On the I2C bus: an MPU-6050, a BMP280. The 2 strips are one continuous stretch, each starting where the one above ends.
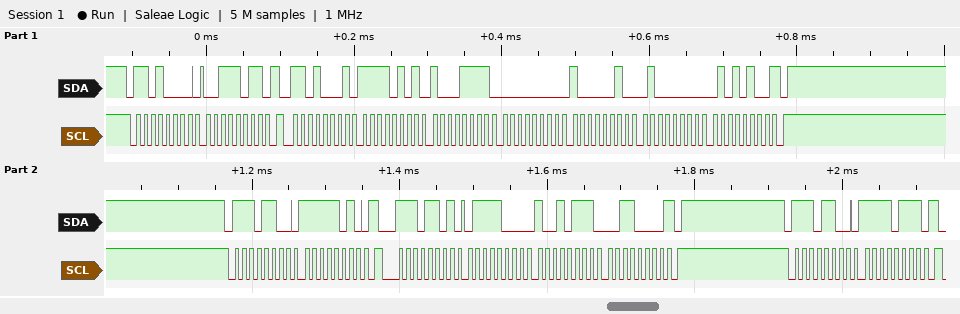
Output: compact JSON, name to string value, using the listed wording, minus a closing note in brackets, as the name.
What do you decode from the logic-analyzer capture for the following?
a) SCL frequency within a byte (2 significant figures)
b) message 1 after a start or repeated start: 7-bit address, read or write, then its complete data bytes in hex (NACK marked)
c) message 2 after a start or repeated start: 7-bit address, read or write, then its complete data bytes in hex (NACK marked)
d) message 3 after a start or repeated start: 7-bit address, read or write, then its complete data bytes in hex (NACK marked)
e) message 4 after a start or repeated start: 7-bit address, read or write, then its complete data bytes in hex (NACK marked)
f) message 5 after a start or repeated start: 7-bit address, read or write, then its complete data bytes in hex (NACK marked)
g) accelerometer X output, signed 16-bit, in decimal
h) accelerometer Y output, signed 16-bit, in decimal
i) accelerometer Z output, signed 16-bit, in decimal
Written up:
{"SCL frequency within a byte": "100 kHz", "message 1 after a start or repeated start: 7-bit address, read or write, then its complete data bytes in hex": "0x68 write: 3B", "message 2 after a start or repeated start: 7-bit address, read or write, then its complete data bytes in hex": "0x68 read: F5 8F 00 82 40 54 NACK", "message 3 after a start or repeated start: 7-bit address, read or write, then its complete data bytes in hex": "0x76 write: FA", "message 4 after a start or repeated start: 7-bit address, read or write, then its complete data bytes in hex": "0x76 read: 78 97 30 NACK", "message 5 after a start or repeated start: 7-bit address, read or write, then its complete data bytes in hex": "0x76 write: F7", "accelerometer X output, signed 16-bit, in decimal": "-2673", "accelerometer Y output, signed 16-bit, in decimal": "130", "accelerometer Z output, signed 16-bit, in decimal": "16468"}
